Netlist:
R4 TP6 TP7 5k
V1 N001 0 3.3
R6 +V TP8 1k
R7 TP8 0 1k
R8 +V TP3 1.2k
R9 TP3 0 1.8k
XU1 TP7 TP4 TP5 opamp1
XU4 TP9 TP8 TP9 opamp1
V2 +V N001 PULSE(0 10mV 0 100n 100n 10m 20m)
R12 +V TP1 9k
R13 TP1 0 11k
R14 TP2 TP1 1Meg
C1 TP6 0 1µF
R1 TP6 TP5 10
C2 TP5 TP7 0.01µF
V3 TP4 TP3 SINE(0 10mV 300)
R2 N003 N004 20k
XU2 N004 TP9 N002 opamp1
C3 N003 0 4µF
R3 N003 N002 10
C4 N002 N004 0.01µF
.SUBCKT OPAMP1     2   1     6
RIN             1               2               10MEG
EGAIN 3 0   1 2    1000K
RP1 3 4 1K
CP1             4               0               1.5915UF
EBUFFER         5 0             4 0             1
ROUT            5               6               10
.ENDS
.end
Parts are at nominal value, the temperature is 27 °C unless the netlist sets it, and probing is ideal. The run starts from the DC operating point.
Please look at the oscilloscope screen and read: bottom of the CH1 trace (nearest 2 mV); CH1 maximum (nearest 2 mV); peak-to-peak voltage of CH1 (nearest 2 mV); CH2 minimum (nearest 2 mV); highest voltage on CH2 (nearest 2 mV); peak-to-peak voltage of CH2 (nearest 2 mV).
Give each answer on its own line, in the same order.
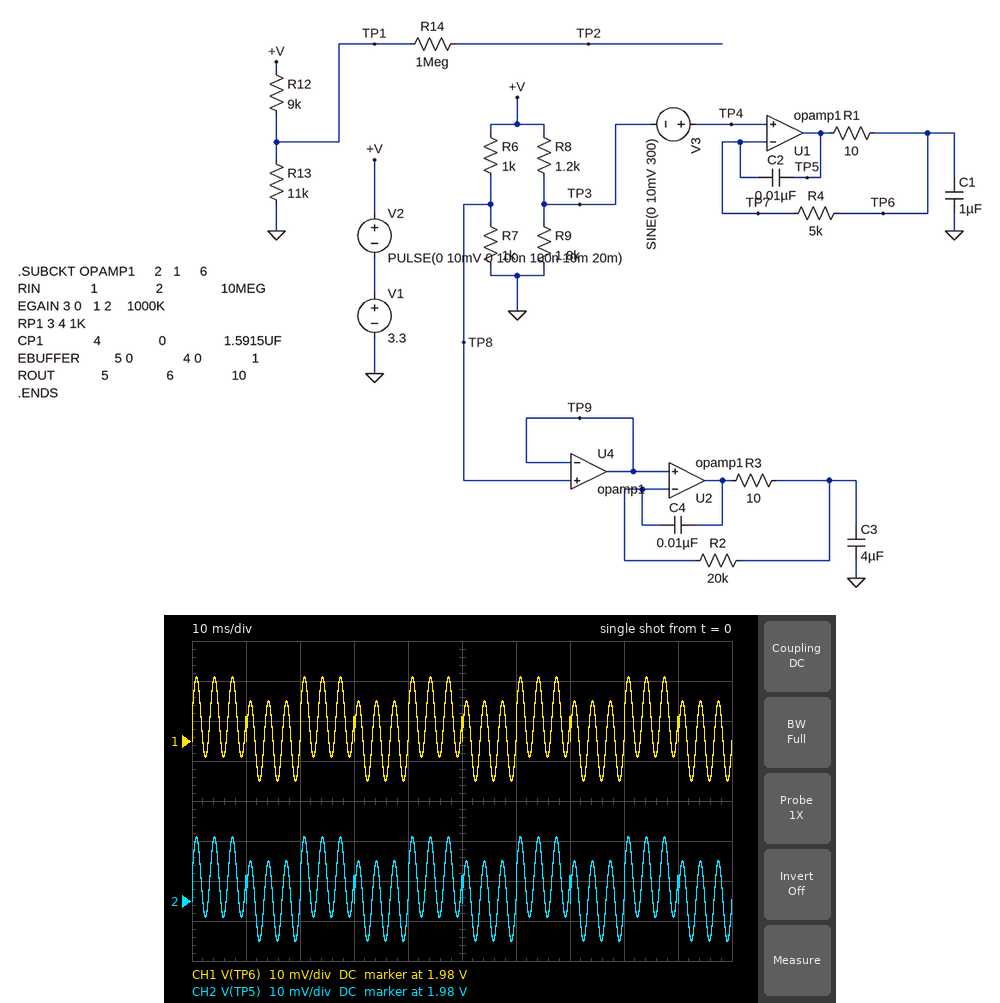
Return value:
1.970 V
1.996 V
26 mV
1.970 V
1.996 V
26 mV
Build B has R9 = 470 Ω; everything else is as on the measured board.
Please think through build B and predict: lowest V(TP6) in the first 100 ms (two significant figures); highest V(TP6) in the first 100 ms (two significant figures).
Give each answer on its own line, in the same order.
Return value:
920 mV
940 mV
